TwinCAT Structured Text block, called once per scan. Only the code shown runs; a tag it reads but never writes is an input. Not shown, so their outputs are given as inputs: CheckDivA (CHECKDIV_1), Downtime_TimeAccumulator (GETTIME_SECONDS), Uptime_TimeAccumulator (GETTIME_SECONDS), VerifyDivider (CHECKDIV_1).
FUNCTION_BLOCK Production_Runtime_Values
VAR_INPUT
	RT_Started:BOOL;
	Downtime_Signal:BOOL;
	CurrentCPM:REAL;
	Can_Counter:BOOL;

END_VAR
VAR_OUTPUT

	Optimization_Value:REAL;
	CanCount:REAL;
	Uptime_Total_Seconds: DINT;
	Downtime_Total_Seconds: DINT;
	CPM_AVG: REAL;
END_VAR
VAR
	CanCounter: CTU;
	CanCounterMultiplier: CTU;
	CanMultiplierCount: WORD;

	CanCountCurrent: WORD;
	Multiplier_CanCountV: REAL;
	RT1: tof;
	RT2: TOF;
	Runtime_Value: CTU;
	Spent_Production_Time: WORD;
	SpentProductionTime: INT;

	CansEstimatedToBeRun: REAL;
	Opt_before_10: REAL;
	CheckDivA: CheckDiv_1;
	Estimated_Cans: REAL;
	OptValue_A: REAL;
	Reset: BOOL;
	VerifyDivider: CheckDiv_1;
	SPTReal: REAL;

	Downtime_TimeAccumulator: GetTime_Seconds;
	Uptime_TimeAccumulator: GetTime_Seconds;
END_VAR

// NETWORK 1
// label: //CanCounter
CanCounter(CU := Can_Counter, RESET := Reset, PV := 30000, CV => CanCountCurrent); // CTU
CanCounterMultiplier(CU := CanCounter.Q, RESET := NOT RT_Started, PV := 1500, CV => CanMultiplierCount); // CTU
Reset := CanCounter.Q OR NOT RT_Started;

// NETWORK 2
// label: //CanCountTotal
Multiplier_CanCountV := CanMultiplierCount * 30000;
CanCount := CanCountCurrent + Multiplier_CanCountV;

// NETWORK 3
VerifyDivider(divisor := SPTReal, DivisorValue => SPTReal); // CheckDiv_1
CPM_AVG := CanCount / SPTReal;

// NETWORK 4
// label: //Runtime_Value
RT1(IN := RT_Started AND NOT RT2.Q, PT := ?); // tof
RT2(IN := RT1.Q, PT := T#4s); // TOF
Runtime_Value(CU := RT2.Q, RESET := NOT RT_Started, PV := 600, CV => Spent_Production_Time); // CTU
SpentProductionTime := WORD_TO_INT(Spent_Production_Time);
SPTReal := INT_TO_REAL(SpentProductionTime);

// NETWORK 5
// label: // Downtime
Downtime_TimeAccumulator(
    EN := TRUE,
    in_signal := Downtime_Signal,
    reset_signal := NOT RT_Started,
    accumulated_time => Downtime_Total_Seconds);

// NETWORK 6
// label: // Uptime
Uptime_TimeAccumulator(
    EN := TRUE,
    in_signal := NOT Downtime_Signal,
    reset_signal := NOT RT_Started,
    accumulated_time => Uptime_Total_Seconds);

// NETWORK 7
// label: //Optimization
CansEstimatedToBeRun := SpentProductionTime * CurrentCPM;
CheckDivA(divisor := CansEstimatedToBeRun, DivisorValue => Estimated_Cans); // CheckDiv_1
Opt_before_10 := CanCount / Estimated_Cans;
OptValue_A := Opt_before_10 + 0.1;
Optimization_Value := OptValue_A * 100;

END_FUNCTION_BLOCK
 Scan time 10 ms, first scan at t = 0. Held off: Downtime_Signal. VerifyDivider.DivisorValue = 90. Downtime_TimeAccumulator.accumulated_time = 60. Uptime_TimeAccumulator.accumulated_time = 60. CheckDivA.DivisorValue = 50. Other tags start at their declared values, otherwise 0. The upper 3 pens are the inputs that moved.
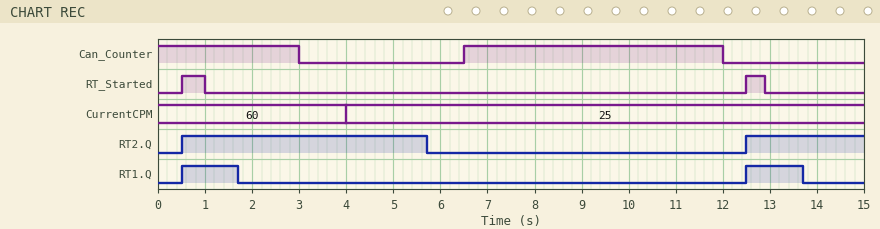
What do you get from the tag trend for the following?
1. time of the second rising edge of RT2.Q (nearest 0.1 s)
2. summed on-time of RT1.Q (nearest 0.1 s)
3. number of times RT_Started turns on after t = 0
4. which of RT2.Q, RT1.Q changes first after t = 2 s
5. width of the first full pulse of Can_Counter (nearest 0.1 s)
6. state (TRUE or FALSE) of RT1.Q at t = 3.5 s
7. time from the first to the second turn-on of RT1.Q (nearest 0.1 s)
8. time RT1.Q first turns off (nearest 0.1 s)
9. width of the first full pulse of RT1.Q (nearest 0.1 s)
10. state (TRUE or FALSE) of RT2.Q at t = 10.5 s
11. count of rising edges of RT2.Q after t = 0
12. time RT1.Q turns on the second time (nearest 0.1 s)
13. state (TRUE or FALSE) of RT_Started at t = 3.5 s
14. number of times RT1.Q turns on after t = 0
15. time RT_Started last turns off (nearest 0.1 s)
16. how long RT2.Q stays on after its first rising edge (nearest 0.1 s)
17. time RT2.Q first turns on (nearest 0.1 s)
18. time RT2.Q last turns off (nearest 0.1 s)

12.5 s
2.4 s
2
RT2.Q
5.5 s
FALSE
12.0 s
1.7 s
1.2 s
FALSE
2
12.5 s
FALSE
2
12.9 s
5.2 s
0.5 s
5.7 s
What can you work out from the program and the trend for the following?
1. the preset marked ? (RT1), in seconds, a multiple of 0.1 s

1.2 s
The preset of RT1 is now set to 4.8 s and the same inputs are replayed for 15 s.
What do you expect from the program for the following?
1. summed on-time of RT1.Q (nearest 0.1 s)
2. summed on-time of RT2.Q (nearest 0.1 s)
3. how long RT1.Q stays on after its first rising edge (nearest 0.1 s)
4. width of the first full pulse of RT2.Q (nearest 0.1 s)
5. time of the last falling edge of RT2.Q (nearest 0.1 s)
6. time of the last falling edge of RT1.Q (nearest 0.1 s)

7.3 s
11.3 s
4.8 s
8.8 s
9.3 s
5.3 s
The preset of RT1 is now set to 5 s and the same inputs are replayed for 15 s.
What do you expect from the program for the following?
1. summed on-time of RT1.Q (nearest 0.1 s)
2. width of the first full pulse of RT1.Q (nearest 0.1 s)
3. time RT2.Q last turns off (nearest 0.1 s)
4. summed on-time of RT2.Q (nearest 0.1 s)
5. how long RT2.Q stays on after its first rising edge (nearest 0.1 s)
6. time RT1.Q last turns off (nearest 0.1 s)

7.5 s
5.0 s
9.5 s
11.5 s
9.0 s
5.5 s
